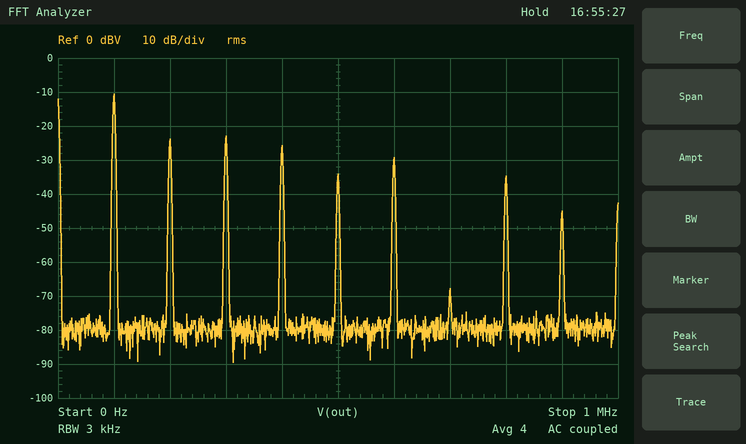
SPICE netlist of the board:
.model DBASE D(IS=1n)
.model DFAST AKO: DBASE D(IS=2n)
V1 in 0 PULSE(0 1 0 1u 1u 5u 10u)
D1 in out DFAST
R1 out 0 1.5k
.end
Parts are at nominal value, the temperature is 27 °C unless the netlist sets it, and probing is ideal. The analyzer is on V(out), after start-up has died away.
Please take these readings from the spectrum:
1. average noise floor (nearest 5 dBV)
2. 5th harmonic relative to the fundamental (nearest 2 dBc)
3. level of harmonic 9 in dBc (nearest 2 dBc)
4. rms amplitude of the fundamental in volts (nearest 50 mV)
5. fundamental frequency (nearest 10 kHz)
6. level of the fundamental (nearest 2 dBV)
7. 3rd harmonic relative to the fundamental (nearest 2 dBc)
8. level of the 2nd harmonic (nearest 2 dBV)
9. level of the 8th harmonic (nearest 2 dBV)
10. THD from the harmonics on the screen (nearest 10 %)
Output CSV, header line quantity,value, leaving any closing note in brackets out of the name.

quantity,value
average noise floor,-80 dBV
5th harmonic relative to the fundamental,-24 dBc
level of harmonic 9 in dBc,-34 dBc
rms amplitude of the fundamental in volts,300 mV
fundamental frequency,100 kHz
level of the fundamental,-10 dBV
3rd harmonic relative to the fundamental,-12 dBc
level of the 2nd harmonic,-24 dBV
level of the 8th harmonic,-34 dBV
THD from the harmonics on the screen,40 %
